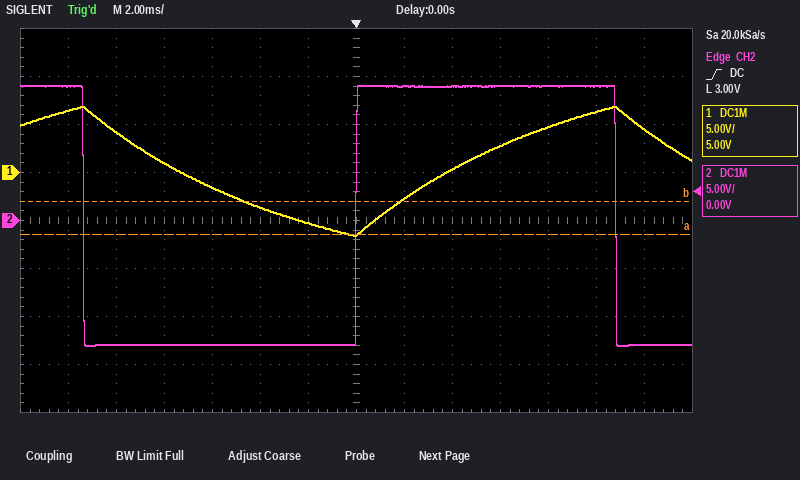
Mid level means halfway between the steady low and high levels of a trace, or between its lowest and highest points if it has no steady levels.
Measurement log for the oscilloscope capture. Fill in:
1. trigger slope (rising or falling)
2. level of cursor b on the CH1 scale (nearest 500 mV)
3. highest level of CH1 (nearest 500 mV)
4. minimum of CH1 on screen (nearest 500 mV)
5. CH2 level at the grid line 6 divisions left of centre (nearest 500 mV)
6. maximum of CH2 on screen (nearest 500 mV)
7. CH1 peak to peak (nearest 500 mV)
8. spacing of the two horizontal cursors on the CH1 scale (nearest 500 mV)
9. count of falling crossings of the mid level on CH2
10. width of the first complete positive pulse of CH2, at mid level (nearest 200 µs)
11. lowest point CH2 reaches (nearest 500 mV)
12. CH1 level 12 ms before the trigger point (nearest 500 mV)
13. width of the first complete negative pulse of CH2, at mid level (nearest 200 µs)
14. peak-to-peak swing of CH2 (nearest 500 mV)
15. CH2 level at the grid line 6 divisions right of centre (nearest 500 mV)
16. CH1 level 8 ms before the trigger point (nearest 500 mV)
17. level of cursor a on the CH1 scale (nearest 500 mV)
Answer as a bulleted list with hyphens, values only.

- rising
- -3.0 V
- 7.0 V
- -6.5 V
- 14.0 V
- 14.0 V
- 13.5 V
- 3.5 V
- 2
- 10.8 ms
- -13.0 V
- 6.5 V
- 11.4 ms
- 27.0 V
- -13.0 V
- 1.0 V
- -6.5 V
